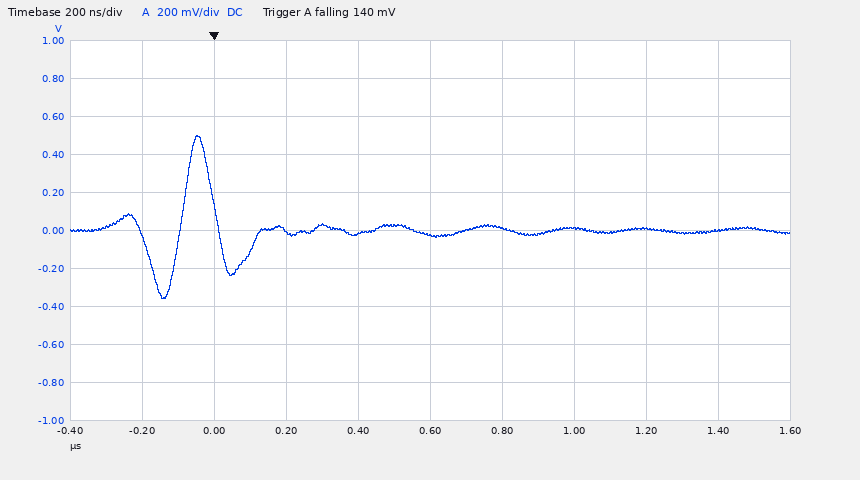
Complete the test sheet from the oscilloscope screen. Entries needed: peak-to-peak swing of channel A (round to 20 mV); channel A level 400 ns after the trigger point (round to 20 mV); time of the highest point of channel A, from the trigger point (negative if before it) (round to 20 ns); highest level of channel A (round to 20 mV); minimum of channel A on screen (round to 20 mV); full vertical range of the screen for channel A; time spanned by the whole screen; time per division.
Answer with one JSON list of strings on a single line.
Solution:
["860 mV", "-20 mV", "-40 ns", "500 mV", "-360 mV", "2 V", "2 µs", "200 ns"]
